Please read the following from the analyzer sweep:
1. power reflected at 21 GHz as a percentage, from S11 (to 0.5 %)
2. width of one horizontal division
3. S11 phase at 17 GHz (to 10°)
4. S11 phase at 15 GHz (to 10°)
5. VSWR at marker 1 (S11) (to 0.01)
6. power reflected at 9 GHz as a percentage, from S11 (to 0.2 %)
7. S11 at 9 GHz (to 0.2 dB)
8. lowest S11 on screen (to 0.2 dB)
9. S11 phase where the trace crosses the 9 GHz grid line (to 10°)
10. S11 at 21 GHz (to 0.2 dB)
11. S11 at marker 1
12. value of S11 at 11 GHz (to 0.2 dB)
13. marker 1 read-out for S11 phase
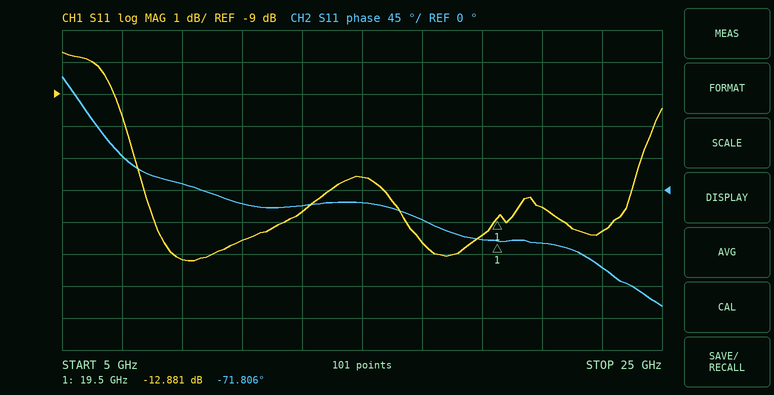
5.5 %
2 GHz
-40°
-20°
1.59
3.8 %
-14.2 dB
-14.2 dB
10°
-12.6 dB
-12.881 dB
-13.6 dB
-71.806°
